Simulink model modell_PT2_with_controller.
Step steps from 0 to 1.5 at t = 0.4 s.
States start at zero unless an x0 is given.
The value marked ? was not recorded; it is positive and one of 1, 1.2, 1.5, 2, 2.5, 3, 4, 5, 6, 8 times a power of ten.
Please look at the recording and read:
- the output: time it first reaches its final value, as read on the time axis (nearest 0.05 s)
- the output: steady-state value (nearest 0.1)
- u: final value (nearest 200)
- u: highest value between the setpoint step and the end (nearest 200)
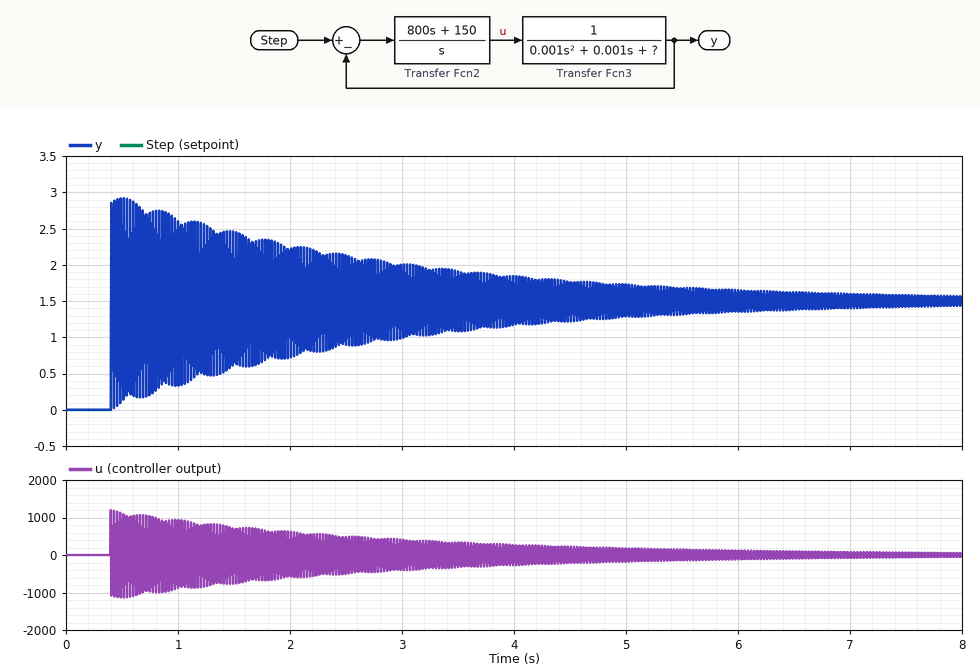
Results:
0.40 s
1.5
0
1200
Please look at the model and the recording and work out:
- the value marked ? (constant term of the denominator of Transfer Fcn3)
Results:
0.6
